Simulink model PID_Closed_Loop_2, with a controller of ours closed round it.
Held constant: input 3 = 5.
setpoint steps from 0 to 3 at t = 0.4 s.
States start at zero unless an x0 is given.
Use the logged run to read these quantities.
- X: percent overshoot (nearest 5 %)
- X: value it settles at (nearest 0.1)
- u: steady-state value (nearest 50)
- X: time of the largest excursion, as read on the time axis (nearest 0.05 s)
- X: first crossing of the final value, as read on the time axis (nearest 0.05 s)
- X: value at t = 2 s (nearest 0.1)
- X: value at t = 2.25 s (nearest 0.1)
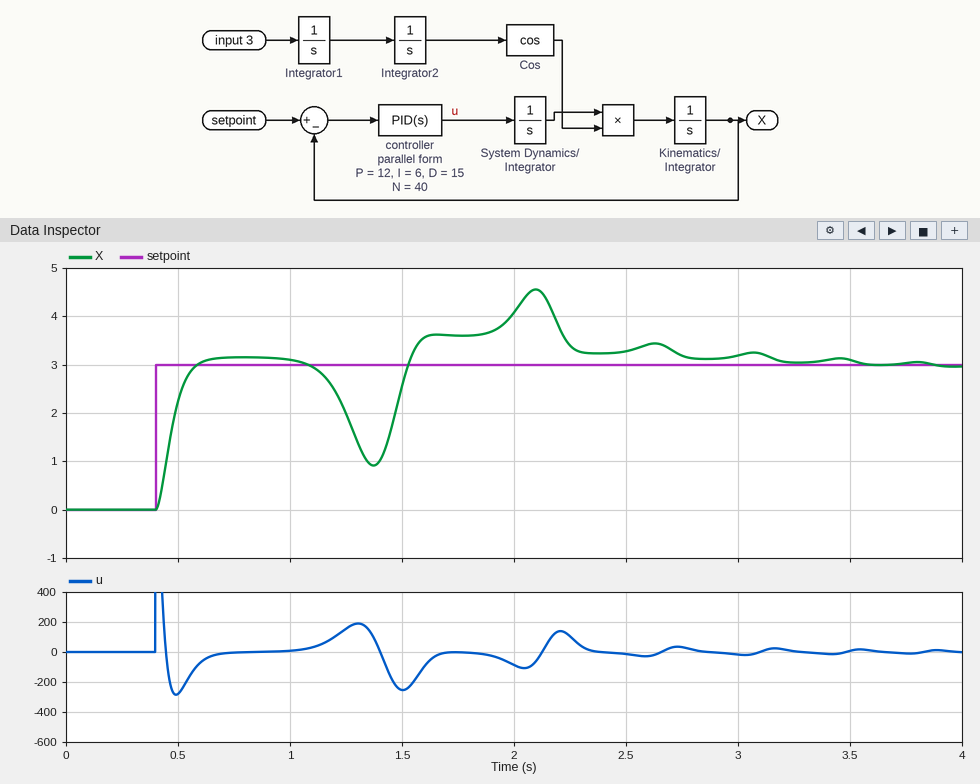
50 %
3.0
0
2.10 s
0.60 s
4.1
3.4
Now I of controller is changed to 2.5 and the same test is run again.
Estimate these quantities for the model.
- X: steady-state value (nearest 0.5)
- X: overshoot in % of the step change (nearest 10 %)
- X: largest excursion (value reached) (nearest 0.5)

3.0
30 %
4.0
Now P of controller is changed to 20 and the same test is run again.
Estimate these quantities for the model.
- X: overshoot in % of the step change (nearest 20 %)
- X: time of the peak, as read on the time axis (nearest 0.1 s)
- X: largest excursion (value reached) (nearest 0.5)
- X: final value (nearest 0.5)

180 %
1.4 s
8.5
3.0
